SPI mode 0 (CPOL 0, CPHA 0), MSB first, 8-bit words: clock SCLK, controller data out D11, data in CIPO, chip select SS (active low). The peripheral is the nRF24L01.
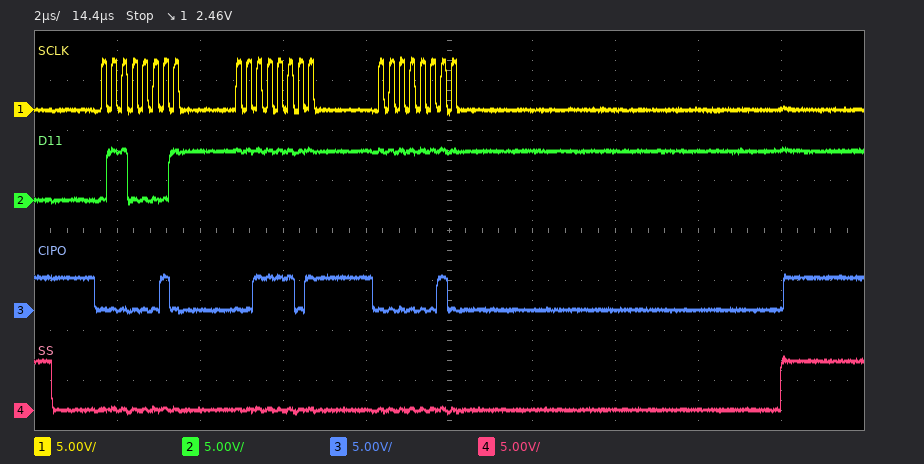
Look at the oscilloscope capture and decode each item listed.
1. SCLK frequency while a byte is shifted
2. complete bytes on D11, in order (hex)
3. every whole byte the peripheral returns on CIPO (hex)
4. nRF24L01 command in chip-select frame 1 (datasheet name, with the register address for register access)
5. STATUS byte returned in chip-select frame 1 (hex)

4 MHz
61 FF FF
02 3D 02
R_RX_PAYLOAD
0x02
